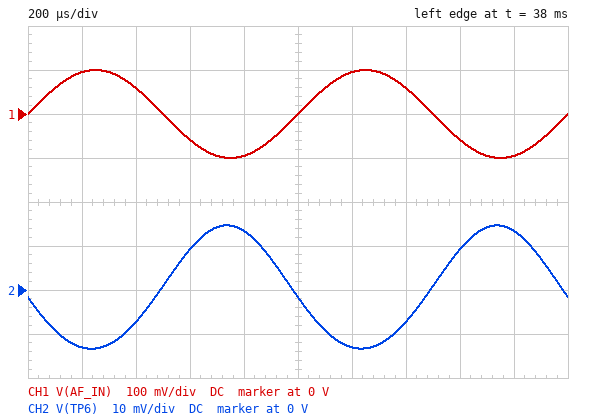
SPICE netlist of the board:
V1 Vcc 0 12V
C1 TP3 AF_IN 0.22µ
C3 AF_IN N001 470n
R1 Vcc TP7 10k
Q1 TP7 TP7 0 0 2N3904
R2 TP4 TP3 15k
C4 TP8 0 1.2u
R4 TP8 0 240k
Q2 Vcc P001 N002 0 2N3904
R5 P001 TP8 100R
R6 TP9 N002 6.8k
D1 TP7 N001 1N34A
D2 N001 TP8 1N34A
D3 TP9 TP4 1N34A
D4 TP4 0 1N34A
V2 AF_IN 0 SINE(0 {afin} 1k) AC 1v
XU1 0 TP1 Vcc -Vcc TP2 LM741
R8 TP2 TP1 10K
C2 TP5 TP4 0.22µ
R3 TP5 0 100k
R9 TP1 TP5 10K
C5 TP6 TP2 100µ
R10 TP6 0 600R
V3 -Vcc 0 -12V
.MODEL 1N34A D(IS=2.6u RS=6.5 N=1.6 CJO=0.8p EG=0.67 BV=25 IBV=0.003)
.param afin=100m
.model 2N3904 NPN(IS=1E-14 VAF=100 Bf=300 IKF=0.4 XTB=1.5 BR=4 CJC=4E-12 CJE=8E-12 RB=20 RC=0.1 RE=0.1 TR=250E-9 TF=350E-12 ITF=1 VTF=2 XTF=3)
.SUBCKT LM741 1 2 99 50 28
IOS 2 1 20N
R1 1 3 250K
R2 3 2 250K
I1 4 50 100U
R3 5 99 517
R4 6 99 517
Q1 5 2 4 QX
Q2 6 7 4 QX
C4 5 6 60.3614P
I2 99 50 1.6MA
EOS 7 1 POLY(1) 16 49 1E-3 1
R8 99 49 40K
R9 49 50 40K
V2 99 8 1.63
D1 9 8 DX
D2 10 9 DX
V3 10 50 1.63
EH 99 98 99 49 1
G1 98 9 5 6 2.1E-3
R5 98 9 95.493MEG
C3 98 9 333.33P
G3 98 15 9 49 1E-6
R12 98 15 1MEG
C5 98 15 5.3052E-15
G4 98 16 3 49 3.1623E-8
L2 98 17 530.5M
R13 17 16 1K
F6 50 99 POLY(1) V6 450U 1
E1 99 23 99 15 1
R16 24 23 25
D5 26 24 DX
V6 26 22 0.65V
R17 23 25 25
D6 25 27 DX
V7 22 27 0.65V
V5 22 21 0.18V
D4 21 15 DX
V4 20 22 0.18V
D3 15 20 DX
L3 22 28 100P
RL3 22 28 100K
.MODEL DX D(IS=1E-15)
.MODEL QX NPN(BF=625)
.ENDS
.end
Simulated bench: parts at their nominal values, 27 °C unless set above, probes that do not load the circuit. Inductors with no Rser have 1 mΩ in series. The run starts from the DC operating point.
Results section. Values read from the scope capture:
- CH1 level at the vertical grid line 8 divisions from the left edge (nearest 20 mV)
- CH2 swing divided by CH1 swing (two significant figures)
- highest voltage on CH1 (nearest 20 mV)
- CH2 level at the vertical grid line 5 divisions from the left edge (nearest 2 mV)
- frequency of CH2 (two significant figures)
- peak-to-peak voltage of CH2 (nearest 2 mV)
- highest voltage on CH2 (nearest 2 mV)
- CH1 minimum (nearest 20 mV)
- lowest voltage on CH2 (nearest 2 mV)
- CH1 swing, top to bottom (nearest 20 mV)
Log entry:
-60 mV
0.14
100 mV
-2 mV
1.0 kHz
28 mV
14 mV
-100 mV
-14 mV
200 mV
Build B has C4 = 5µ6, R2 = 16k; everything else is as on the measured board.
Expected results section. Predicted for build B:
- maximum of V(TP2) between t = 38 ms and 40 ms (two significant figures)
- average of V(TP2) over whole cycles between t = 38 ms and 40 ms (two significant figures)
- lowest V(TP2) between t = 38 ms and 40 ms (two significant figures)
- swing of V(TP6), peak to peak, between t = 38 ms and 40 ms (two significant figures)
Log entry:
17 mV
1.7 mV
-13 mV
30 mV
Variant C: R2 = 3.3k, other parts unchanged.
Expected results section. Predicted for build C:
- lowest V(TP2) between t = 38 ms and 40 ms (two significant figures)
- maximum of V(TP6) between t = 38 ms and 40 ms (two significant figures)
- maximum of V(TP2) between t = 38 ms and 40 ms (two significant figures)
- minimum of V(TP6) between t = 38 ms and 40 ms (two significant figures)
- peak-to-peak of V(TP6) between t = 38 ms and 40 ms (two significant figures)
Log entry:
-38 mV
46 mV
48 mV
-40 mV
86 mV
